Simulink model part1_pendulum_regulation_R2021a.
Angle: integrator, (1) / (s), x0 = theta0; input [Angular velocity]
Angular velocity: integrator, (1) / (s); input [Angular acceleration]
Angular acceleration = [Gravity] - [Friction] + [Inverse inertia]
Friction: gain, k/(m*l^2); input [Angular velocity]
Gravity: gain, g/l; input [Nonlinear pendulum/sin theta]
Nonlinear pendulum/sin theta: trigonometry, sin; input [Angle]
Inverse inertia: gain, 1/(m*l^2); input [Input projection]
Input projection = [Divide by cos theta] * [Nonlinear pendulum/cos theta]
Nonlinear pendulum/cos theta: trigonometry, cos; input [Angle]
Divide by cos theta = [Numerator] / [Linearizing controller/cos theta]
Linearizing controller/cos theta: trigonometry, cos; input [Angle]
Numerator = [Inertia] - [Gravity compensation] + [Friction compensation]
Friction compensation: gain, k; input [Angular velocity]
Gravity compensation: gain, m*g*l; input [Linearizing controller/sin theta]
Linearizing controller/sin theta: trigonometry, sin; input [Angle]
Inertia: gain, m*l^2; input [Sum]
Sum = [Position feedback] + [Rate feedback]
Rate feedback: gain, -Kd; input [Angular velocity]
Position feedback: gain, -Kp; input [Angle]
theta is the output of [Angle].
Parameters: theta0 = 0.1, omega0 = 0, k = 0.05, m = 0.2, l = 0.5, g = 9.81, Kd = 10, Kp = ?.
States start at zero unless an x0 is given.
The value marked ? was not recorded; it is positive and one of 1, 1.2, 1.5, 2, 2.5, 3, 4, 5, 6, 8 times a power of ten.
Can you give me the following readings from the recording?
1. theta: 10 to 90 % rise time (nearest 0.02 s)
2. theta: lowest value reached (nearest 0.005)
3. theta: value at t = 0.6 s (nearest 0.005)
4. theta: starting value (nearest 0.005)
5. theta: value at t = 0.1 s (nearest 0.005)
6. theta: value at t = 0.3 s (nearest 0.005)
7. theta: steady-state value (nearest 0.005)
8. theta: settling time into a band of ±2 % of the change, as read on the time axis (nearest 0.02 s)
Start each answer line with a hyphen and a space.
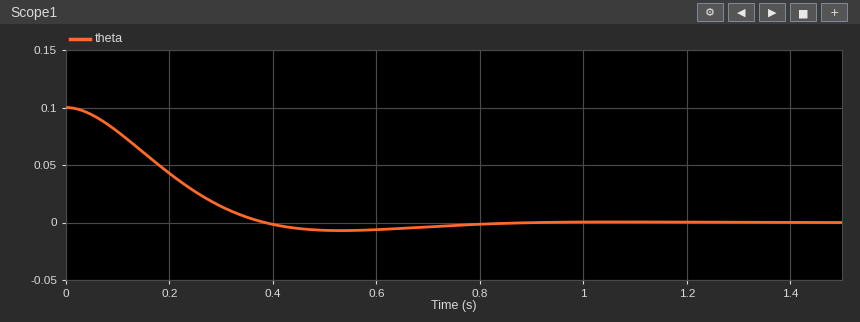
- 0.26 s
- -0.005
- -0.005
- 0.100
- 0.080
- 0.015
- 0.000
- 0.78 s
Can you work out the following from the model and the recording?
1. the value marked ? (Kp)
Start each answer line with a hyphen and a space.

- 60
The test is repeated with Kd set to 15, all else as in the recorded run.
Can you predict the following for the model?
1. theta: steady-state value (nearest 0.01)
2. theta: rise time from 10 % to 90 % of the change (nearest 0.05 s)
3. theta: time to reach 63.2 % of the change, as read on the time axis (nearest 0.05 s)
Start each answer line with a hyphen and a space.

- 0.00
- 0.40 s
- 0.25 s
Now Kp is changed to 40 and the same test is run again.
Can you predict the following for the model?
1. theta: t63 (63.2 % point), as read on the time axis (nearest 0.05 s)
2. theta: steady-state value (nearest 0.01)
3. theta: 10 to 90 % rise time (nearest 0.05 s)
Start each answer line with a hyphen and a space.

- 0.30 s
- 0.00
- 0.40 s
